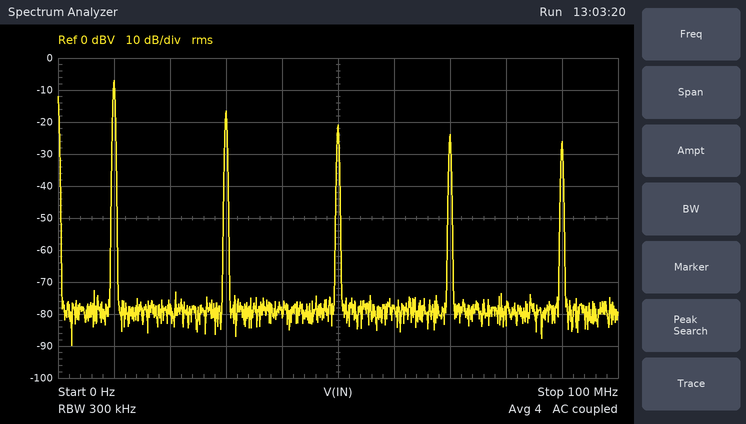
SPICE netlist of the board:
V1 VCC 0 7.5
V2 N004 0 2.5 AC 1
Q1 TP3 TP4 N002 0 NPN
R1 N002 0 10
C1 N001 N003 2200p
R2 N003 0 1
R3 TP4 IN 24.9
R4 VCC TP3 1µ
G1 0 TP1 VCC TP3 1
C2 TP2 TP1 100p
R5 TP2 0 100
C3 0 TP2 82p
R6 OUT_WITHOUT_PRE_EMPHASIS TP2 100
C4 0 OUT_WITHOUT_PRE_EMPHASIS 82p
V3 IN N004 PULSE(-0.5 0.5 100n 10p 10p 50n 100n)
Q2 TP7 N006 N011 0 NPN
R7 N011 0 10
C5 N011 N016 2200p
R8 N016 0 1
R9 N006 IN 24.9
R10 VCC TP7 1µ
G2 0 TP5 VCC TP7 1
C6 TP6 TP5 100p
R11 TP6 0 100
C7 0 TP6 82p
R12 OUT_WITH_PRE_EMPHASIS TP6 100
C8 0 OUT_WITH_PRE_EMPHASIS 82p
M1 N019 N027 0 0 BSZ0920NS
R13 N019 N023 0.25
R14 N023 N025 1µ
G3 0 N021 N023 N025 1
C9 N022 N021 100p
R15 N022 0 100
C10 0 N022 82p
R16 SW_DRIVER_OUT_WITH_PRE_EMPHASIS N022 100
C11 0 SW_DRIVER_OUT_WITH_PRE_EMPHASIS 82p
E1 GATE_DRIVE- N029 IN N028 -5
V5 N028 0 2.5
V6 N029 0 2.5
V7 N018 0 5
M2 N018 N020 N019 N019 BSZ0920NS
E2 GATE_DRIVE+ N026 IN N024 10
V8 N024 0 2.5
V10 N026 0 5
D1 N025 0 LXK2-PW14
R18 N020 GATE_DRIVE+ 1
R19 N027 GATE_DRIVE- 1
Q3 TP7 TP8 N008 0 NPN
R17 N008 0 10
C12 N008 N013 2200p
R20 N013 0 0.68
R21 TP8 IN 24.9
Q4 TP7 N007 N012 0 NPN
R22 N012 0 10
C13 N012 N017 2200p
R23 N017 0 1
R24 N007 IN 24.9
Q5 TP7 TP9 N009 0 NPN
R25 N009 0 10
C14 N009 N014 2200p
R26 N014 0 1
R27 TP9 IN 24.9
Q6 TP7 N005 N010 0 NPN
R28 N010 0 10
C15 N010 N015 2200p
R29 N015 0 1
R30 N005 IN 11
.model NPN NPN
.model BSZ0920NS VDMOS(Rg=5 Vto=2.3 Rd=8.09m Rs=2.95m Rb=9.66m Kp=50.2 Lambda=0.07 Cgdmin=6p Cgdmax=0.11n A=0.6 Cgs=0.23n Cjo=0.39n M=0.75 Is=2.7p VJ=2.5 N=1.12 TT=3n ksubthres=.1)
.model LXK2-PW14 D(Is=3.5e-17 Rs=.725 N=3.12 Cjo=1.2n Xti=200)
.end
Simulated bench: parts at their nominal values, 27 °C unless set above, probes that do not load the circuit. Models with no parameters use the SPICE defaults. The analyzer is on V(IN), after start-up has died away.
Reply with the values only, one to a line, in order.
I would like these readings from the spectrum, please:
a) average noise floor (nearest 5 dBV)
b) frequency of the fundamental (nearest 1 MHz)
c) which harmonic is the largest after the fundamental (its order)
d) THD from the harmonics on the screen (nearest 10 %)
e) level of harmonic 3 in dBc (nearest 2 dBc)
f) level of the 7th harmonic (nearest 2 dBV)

-80 dBV
10 MHz
3
40 %
-10 dBc
-24 dBV
